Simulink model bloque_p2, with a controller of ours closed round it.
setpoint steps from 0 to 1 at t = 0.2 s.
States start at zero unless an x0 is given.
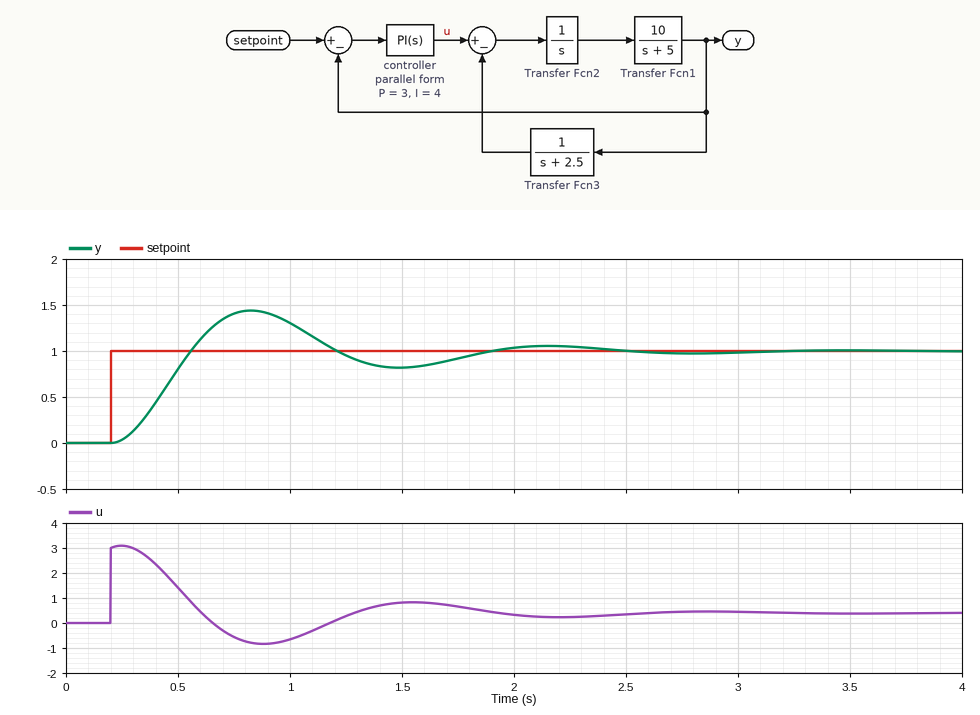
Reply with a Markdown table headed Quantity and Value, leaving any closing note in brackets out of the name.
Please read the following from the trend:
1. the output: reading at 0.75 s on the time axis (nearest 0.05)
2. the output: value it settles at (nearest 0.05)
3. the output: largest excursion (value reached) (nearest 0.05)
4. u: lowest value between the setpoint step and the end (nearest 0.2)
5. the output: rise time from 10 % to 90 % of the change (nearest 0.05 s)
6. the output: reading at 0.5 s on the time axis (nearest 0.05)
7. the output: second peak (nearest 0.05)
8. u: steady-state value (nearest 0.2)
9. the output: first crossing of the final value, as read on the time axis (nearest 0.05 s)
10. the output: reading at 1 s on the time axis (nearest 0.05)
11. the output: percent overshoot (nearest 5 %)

| Quantity | Value |
|---|---|
| the output: reading at 0.75 s on the time axis | 1.40 |
| the output: value it settles at | 1.00 |
| the output: largest excursion (value reached) | 1.45 |
| u: lowest value between the setpoint step and the end | -0.8 |
| the output: rise time from 10 % to 90 % of the change | 0.25 s |
| the output: reading at 0.5 s on the time axis | 0.80 |
| the output: second peak | 1.05 |
| u: steady-state value | 0.4 |
| the output: first crossing of the final value, as read on the time axis | 0.55 s |
| the output: reading at 1 s on the time axis | 1.30 |
| the output: percent overshoot | 45 % |
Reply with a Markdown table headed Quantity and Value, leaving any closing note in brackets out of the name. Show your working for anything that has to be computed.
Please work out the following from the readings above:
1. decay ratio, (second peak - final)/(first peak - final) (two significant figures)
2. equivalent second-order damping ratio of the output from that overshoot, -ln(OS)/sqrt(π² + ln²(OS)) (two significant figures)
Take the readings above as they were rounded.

| Quantity | Value |
|---|---|
| decay ratio, (second peak - final)/(first peak - final) | (1.05 - 1) / (1.45 - 1) = 0.11 |
| equivalent second-order damping ratio of the output from that overshoot, -ln(OS)/sqrt(π² + ln²(OS)) | ln(0.45) = -0.799; 0.799 / sqrt(9.870 + 0.638) = 0.25 |
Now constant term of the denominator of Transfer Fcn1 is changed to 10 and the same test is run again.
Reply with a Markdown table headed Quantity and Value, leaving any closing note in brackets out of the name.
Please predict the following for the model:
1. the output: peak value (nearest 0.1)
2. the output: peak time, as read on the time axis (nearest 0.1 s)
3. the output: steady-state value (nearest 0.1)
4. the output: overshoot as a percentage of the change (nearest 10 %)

| Quantity | Value |
|---|---|
| the output: peak value | 1.2 |
| the output: peak time, as read on the time axis | 1.1 s |
| the output: steady-state value | 1.0 |
| the output: overshoot as a percentage of the change | 20 % |
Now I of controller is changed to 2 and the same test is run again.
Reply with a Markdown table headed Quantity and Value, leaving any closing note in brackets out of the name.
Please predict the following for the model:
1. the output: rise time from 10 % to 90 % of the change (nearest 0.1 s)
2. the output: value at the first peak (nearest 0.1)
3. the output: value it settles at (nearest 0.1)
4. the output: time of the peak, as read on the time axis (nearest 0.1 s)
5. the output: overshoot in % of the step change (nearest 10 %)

| Quantity | Value |
|---|---|
| the output: rise time from 10 % to 90 % of the change | 0.3 s |
| the output: value at the first peak | 1.3 |
| the output: value it settles at | 1.0 |
| the output: time of the peak, as read on the time axis | 0.8 s |
| the output: overshoot in % of the step change | 30 % |
